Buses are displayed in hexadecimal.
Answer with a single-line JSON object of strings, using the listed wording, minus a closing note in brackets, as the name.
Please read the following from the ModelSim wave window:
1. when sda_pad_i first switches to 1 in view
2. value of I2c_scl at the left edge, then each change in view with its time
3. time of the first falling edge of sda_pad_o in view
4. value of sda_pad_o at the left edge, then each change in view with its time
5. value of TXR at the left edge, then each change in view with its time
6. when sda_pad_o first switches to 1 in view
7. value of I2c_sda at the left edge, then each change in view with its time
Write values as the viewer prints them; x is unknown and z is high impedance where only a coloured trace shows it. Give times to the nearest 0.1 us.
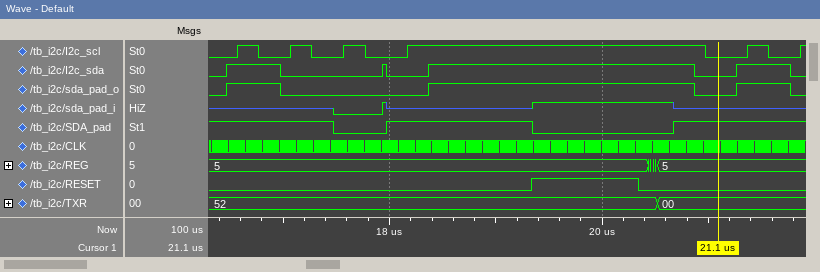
{"when sda_pad_i first switches to 1 in view": "17.9 us", "value of I2c_scl at the left edge, then each change in view with its time": "0, 1 at 16.6 us, 0 at 16.8 us, 1 at 17.1 us, 0 at 17.3 us, 1 at 17.6 us, 0 at 17.8 us, 1 at 18.2 us, 0 at 21 us, 1 at 21.4 us, 0 at 21.6 us, 1 at 21.9 us", "time of the first falling edge of sda_pad_o in view": "17 us", "value of sda_pad_o at the left edge, then each change in view with its time": "0, 1 at 16.5 us, 0 at 17 us, 1 at 18.4 us, 0 at 20.9 us, 1 at 21.3 us, 0 at 21.8 us", "value of TXR at the left edge, then each change in view with its time": "52, 00 at 20.5 us", "when sda_pad_o first switches to 1 in view": "16.5 us", "value of I2c_sda at the left edge, then each change in view with its time": "0, 1 at 16.5 us, 0 at 17 us, 1 at 17.9 us, 0 at 18 us, 1 at 18.4 us, 0 at 20.9 us, 1 at 21.3 us, 0 at 21.8 us"}
